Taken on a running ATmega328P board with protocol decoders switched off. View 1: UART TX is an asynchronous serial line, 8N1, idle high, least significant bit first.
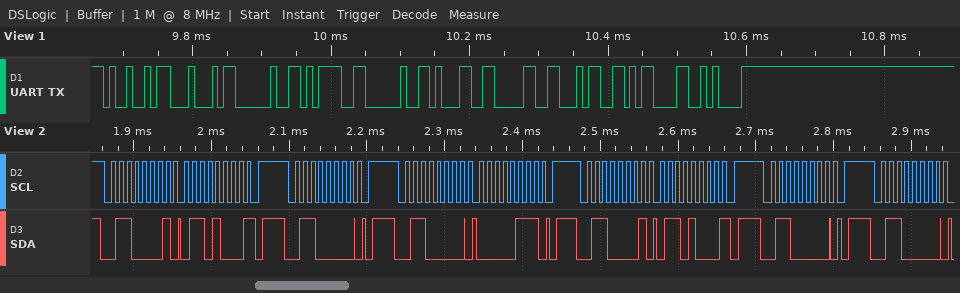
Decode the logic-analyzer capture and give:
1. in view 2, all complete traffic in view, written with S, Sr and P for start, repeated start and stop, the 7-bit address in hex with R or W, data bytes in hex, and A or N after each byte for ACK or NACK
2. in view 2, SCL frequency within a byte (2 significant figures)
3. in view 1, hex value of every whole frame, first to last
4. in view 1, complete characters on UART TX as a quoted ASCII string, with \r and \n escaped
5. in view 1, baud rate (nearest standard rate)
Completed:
S 30R A 68 N P S 30W A P S 30W A 07 A P S 30R A 68 N P S 30W A P S 30W A
100 kHz
49 44 20 3D 20 31 30 34 0D 0A
"ID = 104\r\n"
115200 baud
